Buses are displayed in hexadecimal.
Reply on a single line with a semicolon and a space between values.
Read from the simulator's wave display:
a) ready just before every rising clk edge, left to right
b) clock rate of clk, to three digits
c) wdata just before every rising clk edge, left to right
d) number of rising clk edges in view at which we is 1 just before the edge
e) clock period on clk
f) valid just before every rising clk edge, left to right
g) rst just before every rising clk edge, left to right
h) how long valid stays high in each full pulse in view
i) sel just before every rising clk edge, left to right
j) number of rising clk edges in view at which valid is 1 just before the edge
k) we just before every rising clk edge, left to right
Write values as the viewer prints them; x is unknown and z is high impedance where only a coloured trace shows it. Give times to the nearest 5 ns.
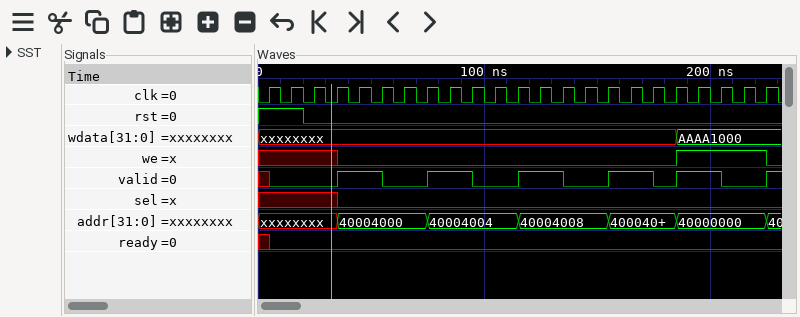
x 0 0 0 0 0 0 0 0 0 0 0 0 0 0 0 0 0 0 0 0 0 0; 100 MHz; xxxxxxxx, xxxxxxxx, xxxxxxxx, xxxxxxxx, xxxxxxxx, xxxxxxxx, xxxxxxxx, xxxxxxxx, xxxxxxxx, xxxxxxxx, xxxxxxxx, xxxxxxxx, xxxxxxxx, xxxxxxxx, xxxxxxxx, xxxxxxxx, xxxxxxxx, xxxxxxxx, xxxxxxxx, AAAA1000, AAAA1000, AAAA1000, AAAA1000; 4; 10 ns; x 0 0 0 1 1 0 0 1 1 0 0 1 1 0 0 1 1 0 1 1 0 0; 1 1 0 0 0 0 0 0 0 0 0 0 0 0 0 0 0 0 0 0 0 0 0; 20 ns, 20 ns, 20 ns, 20 ns, 20 ns; x x x x 0 0 0 0 0 0 0 0 0 0 0 0 0 0 0 0 0 0 0; 10; x x x x 0 0 0 0 0 0 0 0 0 0 0 0 0 0 0 1 1 1 1
